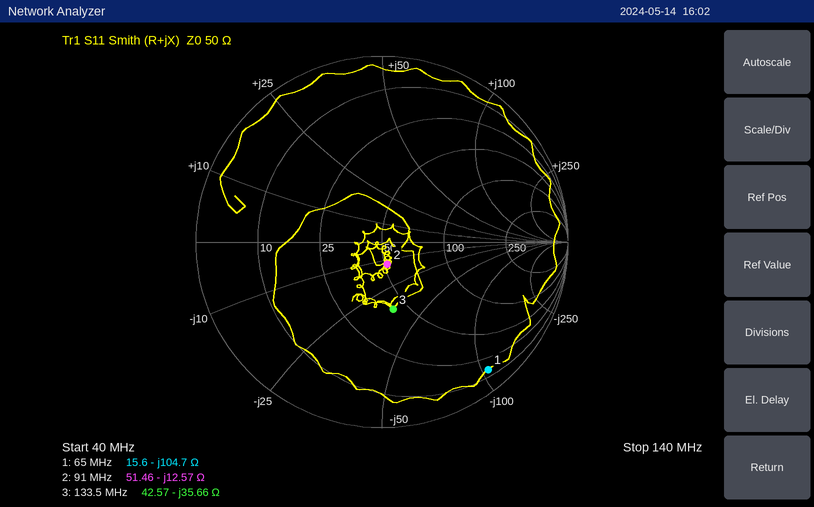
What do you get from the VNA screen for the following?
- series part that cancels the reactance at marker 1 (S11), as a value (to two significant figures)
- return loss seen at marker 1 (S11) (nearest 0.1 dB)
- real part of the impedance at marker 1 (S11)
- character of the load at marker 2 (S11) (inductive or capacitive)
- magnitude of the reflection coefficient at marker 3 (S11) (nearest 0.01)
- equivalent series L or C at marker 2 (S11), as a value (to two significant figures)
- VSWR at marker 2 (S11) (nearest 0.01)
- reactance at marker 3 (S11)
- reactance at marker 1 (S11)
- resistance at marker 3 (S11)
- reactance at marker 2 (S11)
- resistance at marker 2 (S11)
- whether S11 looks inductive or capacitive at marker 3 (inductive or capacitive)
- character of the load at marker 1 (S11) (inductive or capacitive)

260 nH
1.0 dB
15.6 Ω
capacitive
0.37
140 pF
1.28
-35.66 Ω
-104.7 Ω
42.57 Ω
-12.57 Ω
51.46 Ω
capacitive
capacitive
